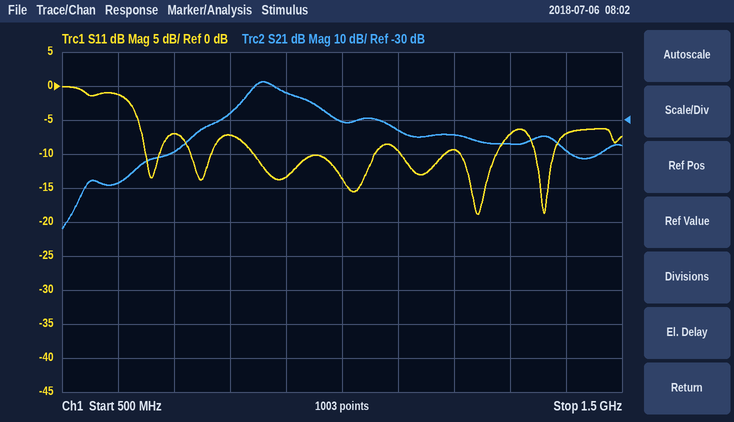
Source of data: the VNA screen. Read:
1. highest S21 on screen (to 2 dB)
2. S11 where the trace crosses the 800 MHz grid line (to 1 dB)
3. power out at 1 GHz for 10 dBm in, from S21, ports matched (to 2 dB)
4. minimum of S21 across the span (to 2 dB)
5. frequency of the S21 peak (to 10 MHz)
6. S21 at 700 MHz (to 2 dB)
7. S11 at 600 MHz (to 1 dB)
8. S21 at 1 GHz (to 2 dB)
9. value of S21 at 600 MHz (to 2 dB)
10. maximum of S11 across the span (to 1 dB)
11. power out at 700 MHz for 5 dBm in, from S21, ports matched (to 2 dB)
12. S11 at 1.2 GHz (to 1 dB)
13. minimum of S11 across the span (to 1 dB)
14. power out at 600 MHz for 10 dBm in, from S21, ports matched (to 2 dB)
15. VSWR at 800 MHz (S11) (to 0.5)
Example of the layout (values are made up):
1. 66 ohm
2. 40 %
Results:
1. -18 dB
2. -7 dB
3. -20 dBm
4. -62 dB
5. 860 MHz
6. -40 dB
7. -1 dB
8. -30 dB
9. -48 dB
10. 0 dB
11. -34 dBm
12. -9 dB
13. -19 dB
14. -38 dBm
15. 2.5
